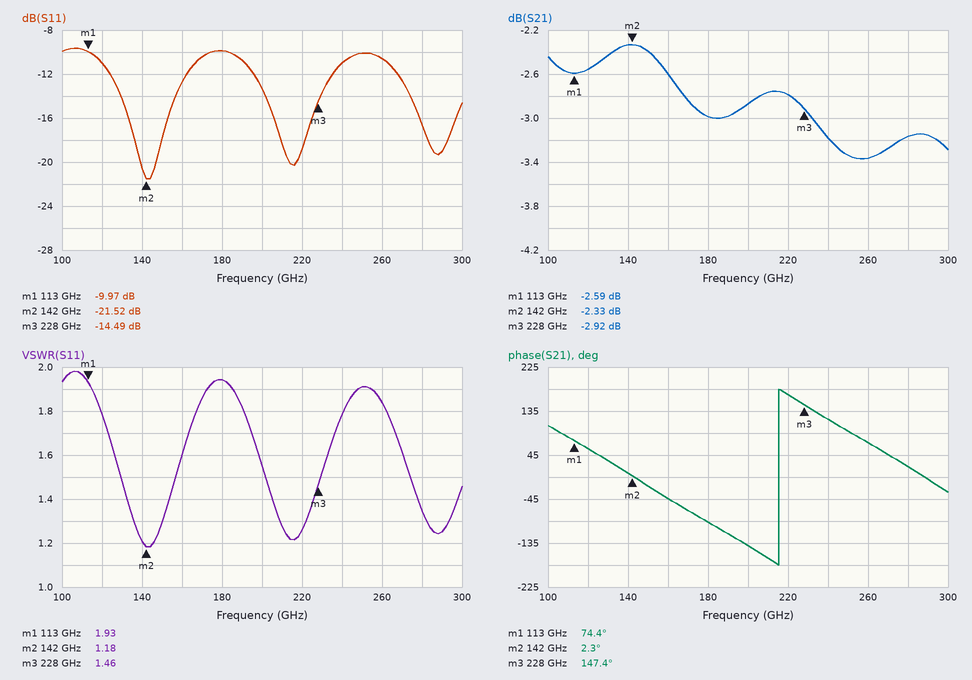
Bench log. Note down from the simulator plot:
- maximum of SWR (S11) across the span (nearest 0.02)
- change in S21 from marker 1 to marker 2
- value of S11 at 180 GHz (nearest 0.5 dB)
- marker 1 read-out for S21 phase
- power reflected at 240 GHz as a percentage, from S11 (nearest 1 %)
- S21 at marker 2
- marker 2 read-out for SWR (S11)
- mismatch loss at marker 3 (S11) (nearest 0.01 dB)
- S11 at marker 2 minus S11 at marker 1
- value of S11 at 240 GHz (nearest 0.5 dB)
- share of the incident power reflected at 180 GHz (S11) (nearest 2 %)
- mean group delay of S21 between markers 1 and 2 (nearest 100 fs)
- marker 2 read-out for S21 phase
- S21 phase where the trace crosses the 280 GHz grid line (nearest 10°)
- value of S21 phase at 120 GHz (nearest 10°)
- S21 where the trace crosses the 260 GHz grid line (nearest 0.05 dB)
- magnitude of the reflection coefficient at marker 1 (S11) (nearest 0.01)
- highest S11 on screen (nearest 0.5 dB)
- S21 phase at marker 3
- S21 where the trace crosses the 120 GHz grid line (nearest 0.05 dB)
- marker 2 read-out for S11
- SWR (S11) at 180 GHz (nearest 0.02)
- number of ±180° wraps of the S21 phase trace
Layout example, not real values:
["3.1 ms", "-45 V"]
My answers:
["1.98", "0.26 dB", "-10.0 dB", "74.4°", "8 %", "-2.33 dB", "1.18", "0.16 dB", "-11.55 dB", "-11.0 dB", "10 %", "6.9 ps", "2.3°", "20°", "60°", "-3.35 dB", "0.32", "-9.5 dB", "147.4°", "-2.55 dB", "-21.52 dB", "1.94", "1"]
